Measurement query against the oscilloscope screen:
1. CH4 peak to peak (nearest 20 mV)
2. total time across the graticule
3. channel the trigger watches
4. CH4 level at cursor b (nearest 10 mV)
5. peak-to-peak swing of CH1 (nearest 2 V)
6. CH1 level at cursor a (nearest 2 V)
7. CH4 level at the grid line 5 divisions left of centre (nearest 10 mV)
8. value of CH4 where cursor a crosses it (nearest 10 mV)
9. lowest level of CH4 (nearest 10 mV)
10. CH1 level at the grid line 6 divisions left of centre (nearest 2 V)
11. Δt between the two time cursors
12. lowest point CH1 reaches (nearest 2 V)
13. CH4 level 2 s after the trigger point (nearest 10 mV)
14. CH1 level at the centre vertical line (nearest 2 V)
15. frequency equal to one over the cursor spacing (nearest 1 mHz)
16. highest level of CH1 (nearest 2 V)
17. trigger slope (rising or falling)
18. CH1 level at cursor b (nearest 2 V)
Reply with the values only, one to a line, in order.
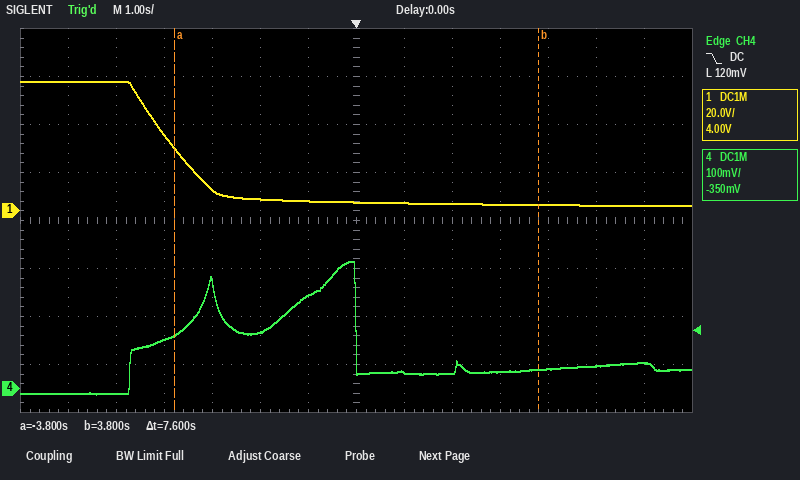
280 mV
14 s
CH4
40 mV
52 V
26 V
-10 mV
110 mV
-10 mV
54 V
7.6 s
2 V
30 mV
4 V
132 mHz
54 V
falling
2 V
